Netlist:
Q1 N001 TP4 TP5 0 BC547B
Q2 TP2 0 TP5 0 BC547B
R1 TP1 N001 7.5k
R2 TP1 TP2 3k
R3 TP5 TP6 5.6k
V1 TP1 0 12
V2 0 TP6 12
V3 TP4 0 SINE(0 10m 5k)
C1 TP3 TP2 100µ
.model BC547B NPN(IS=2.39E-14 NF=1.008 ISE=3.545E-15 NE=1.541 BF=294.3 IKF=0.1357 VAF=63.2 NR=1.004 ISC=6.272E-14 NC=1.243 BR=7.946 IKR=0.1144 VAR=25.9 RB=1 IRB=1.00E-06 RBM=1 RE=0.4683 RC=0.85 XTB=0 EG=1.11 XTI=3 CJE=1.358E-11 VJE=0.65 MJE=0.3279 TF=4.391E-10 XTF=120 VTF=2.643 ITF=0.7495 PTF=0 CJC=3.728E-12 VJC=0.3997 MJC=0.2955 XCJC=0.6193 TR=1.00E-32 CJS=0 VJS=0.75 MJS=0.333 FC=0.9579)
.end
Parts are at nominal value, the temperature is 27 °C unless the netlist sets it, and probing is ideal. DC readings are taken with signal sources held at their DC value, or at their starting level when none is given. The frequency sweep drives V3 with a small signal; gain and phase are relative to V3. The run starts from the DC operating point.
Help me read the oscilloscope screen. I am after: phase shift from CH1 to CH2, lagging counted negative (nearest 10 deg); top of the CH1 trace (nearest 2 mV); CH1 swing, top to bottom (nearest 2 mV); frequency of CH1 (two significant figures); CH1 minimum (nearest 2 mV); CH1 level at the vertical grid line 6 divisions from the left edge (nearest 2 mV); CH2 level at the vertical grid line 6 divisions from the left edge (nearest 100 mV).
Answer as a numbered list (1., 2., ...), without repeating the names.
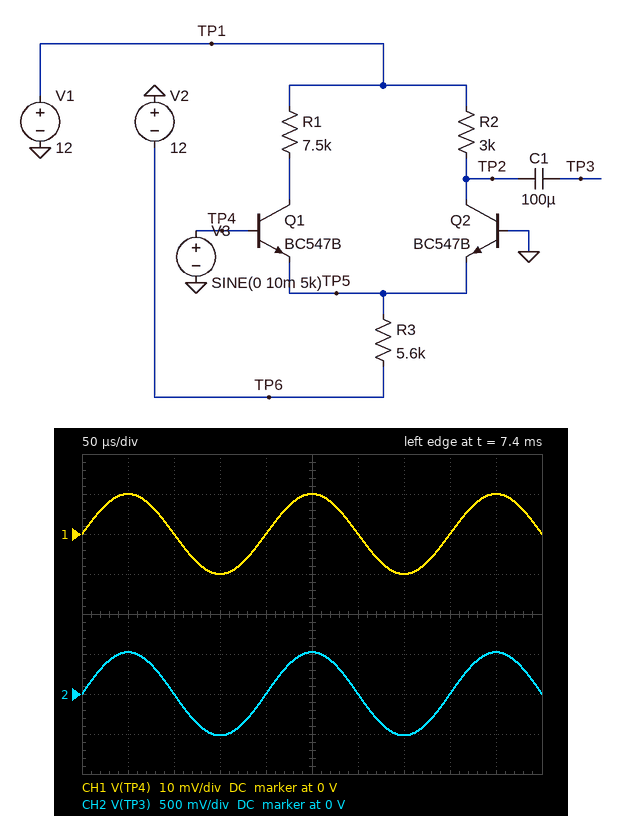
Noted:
1. 0 deg
2. 10 mV
3. 20 mV
4. 5.0 kHz
5. -10 mV
6. 0 V
7. 0 V
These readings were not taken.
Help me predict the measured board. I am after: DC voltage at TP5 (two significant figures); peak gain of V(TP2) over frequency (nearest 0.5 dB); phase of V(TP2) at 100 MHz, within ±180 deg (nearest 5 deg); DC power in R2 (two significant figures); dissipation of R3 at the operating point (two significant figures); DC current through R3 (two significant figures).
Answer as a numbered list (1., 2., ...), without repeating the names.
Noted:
1. -640 mV
2. 34.5 dB
3. -70 deg
4. 3.3 mW
5. 23 mW
6. 2.0 mA
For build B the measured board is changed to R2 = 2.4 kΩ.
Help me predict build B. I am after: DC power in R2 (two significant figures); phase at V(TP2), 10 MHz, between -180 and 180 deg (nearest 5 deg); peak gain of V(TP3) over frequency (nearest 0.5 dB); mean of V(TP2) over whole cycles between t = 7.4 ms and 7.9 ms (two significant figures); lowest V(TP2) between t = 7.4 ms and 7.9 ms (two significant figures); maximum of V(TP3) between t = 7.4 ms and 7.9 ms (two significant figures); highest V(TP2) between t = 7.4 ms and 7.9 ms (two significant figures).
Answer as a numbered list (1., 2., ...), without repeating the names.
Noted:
1. 2.6 mW
2. -10 deg
3. 32.5 dB
4. 9.5 V
5. 9.1 V
6. 420 mV
7. 9.9 V
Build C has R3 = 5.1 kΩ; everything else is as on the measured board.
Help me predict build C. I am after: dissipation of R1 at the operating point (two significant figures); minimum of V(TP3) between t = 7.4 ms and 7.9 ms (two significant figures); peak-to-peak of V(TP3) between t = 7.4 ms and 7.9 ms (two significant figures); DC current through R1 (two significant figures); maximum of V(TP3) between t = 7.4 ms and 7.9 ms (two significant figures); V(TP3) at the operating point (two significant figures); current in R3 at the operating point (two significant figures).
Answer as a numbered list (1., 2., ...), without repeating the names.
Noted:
1. 8.6 mW
2. -560 mV
3. 1.1 V
4. 1.1 mA
5. 570 mV
6. 8.6 V
7. 2.2 mA
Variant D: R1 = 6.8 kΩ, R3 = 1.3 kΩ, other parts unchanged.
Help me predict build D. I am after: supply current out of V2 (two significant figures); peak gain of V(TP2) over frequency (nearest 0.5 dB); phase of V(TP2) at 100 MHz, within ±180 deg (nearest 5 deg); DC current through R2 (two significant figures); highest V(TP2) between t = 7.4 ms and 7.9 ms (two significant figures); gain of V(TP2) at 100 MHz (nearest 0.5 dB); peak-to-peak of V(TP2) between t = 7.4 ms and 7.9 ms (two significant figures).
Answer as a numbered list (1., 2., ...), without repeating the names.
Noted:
1. 8.7 mA
2. -3.0 dB
3. -15 deg
4. 4.2 mA
5. -680 mV
6. -3.5 dB
7. 14 mV
